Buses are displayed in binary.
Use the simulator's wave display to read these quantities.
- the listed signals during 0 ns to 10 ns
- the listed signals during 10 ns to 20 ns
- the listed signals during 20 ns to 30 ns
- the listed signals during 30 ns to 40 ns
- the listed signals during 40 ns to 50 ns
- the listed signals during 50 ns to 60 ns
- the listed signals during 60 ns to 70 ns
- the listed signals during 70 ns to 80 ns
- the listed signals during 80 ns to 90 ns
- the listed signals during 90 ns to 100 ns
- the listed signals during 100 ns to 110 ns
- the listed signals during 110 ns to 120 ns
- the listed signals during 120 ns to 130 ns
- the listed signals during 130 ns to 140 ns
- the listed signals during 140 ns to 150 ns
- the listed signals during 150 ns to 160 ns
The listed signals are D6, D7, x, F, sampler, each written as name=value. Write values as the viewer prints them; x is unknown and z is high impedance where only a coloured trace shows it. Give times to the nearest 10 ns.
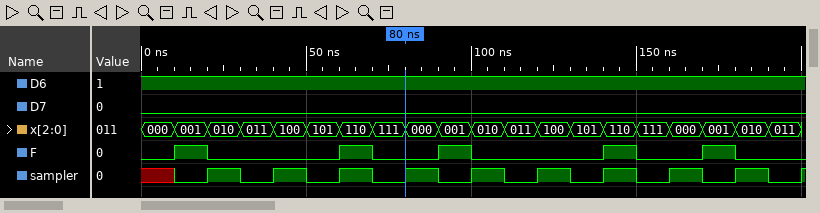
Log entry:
D6=1, D7=0, x=000, F=0, sampler=x
D6=1, D7=0, x=001, F=1, sampler=0
D6=1, D7=0, x=010, F=0, sampler=1
D6=1, D7=0, x=011, F=0, sampler=0
D6=1, D7=0, x=100, F=0, sampler=1
D6=1, D7=0, x=101, F=0, sampler=0
D6=1, D7=0, x=110, F=1, sampler=1
D6=1, D7=0, x=111, F=0, sampler=0
D6=1, D7=0, x=000, F=0, sampler=1
D6=1, D7=0, x=001, F=1, sampler=0
D6=1, D7=0, x=010, F=0, sampler=1
D6=1, D7=0, x=011, F=0, sampler=0
D6=1, D7=0, x=100, F=0, sampler=1
D6=1, D7=0, x=101, F=0, sampler=0
D6=1, D7=0, x=110, F=1, sampler=1
D6=1, D7=0, x=111, F=0, sampler=0
